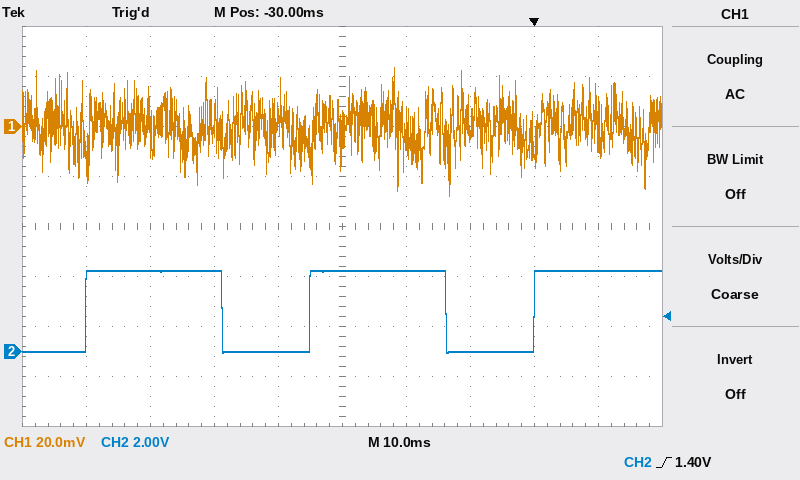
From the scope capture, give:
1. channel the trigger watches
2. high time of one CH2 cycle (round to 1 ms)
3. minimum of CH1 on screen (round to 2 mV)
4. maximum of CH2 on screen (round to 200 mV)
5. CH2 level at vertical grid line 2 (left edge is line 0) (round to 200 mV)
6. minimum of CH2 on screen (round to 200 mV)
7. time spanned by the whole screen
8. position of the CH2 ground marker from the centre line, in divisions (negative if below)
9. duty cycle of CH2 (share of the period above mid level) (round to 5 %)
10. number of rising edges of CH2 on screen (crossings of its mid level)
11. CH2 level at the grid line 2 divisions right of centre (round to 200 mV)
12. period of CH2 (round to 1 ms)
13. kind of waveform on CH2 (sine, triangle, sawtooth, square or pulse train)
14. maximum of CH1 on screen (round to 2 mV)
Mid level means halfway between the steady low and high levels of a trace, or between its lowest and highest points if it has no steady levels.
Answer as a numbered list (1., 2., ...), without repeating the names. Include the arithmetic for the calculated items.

1. CH2
2. 21 ms
3. -28 mV
4. 3.2 V
5. 3.2 V
6. 0.0 V
7. 100 ms
8. -2.5 div
9. 21 ms / 35 ms ≈ 60 %
10. 3
11. 0.0 V
12. 35 ms
13. pulse train
14. 24 mV
